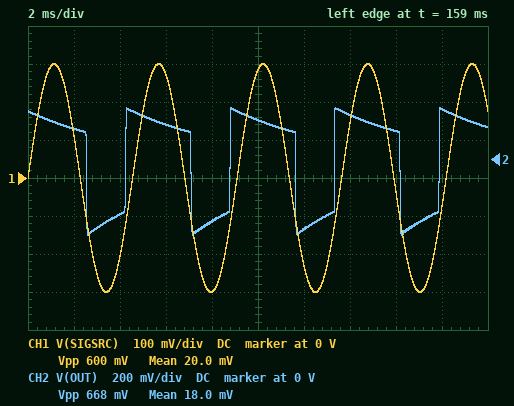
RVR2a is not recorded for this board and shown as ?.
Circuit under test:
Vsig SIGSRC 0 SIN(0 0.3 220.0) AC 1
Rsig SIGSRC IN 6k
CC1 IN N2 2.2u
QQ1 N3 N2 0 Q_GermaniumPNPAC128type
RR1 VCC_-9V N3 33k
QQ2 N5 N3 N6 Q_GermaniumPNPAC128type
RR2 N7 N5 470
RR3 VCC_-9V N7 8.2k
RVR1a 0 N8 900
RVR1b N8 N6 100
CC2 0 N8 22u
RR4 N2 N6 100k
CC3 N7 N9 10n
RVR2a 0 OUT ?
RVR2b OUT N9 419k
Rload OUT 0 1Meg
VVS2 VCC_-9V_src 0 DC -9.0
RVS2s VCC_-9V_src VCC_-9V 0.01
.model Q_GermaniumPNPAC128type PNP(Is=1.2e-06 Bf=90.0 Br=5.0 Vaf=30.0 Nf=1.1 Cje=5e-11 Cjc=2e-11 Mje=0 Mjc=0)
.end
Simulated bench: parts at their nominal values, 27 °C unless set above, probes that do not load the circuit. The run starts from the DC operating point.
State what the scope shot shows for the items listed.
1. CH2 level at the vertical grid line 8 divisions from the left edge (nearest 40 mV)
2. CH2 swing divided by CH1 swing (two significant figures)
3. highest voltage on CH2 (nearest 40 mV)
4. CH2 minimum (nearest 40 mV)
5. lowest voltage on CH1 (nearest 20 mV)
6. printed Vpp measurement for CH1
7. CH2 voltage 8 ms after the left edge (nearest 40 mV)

160 mV
1.1
280 mV
-400 mV
-300 mV
600 mV
-320 mV
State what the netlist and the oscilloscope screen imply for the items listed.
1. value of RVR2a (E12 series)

33 kΩ
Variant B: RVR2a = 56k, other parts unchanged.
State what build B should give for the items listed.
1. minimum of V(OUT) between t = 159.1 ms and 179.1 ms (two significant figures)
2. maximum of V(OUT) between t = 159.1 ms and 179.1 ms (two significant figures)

-630 mV
420 mV
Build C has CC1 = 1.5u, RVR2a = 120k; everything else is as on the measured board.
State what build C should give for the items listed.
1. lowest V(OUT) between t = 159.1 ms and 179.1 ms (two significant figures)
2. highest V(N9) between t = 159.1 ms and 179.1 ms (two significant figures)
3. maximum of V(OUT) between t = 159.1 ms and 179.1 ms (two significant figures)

-1.1 V
3.6 V
740 mV
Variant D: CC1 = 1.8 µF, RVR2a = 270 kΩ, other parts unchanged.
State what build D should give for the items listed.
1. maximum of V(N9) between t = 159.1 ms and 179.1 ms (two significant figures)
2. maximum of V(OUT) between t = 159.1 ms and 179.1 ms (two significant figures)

3.5 V
1.2 V
